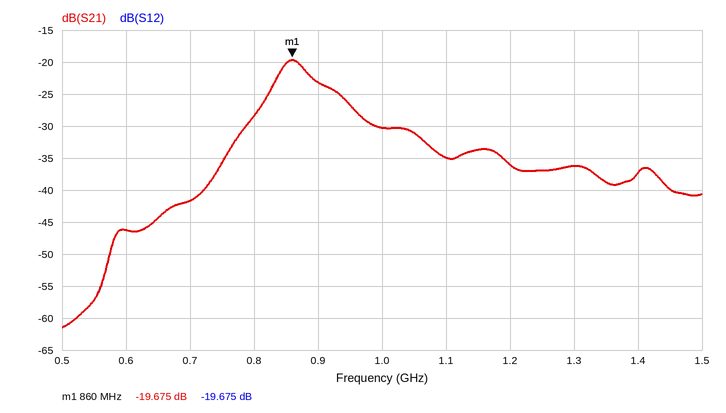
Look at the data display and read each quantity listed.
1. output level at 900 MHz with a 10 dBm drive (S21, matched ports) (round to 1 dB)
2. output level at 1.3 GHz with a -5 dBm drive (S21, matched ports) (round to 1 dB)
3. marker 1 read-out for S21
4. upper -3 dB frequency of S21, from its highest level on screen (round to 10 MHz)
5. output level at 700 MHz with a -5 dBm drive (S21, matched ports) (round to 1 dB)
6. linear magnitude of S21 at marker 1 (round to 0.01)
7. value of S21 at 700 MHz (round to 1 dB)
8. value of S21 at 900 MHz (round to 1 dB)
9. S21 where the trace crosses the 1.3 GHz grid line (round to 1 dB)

-13 dBm
-41 dBm
-19.675 dB
890 MHz
-47 dBm
0.10
-42 dB
-23 dB
-36 dB
